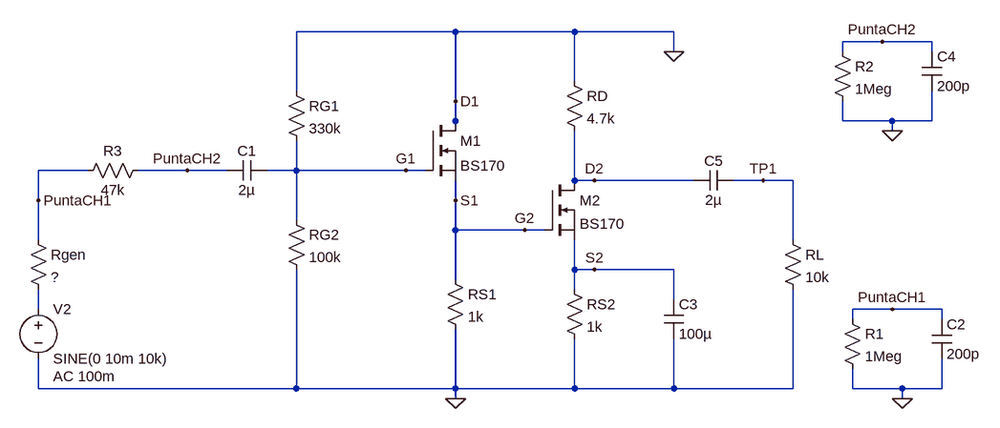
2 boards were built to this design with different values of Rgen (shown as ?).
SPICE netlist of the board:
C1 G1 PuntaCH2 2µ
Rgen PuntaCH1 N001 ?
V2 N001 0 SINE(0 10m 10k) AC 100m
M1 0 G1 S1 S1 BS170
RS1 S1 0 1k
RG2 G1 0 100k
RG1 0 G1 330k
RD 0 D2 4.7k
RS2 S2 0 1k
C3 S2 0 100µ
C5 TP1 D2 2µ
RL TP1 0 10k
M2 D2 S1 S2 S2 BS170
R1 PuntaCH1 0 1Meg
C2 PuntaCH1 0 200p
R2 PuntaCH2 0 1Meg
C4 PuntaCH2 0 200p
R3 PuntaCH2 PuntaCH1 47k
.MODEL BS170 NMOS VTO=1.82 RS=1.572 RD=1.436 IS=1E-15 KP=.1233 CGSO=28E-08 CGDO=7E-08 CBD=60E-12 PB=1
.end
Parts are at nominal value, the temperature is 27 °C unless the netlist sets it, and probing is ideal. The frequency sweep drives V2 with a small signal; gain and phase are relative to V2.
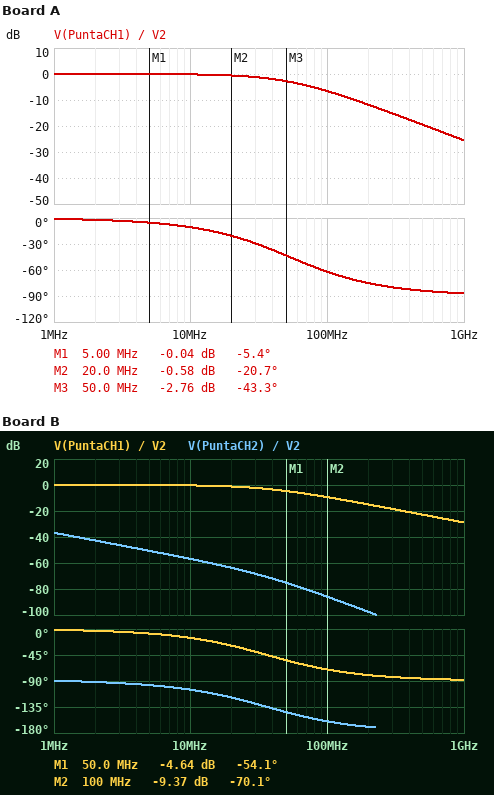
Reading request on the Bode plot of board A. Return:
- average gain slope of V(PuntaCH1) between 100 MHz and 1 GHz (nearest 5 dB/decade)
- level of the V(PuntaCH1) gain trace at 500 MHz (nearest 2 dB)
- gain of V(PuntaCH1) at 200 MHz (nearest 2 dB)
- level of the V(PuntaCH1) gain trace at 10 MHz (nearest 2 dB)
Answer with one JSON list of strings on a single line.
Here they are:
["-20 dB/decade", "-20 dB", "-12 dB", "0 dB"]
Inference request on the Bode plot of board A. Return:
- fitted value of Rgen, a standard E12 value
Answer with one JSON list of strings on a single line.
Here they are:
["15 Ω"]
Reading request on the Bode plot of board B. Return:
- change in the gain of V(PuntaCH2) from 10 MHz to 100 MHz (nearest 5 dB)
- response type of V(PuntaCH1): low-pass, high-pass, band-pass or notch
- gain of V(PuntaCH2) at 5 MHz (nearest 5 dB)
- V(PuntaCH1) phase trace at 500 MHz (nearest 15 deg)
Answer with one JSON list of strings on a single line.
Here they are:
["-30 dB", "low-pass", "-50 dB", "-90 deg"]
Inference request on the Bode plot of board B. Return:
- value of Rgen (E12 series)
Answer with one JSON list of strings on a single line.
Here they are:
["22 Ω"]
